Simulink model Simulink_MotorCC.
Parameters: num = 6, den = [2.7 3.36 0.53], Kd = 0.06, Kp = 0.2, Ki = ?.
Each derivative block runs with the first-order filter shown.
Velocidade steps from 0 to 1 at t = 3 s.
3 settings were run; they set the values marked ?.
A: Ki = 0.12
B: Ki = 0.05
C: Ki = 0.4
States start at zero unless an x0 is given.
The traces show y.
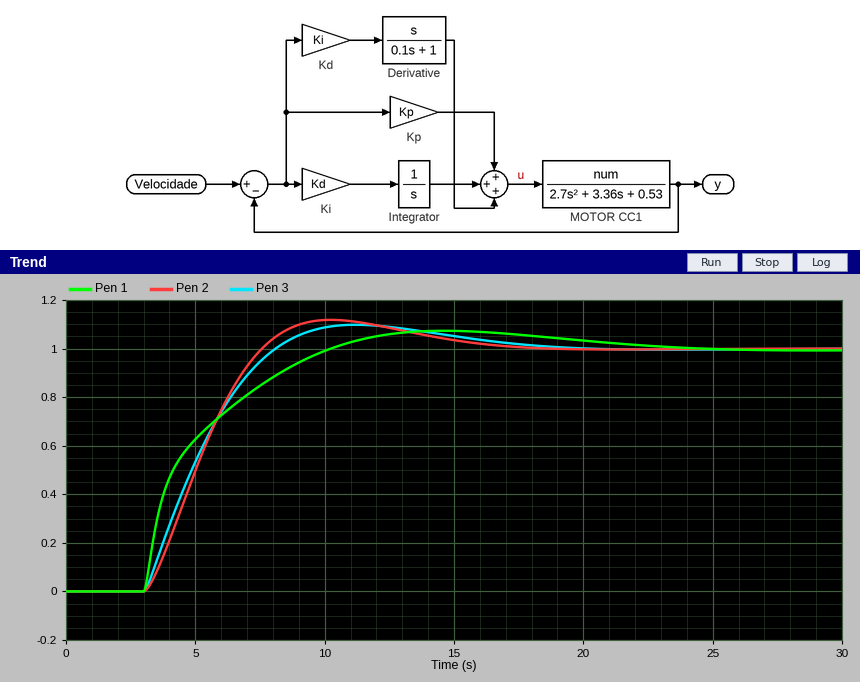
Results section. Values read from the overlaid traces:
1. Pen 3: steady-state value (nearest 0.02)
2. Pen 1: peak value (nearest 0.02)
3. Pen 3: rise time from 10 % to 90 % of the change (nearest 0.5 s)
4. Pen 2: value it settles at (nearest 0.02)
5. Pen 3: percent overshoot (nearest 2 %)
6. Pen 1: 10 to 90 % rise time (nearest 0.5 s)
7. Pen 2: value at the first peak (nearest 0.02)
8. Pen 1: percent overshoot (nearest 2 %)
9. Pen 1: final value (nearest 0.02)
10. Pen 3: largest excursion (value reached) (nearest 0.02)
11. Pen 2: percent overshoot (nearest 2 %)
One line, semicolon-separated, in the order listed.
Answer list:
1.00; 1.08; 3.5 s; 1.00; 10 %; 5.0 s; 1.12; 8 %; 1.00; 1.10; 12 %
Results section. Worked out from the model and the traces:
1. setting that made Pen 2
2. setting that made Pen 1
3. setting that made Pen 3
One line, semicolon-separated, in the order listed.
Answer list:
B; C; A
